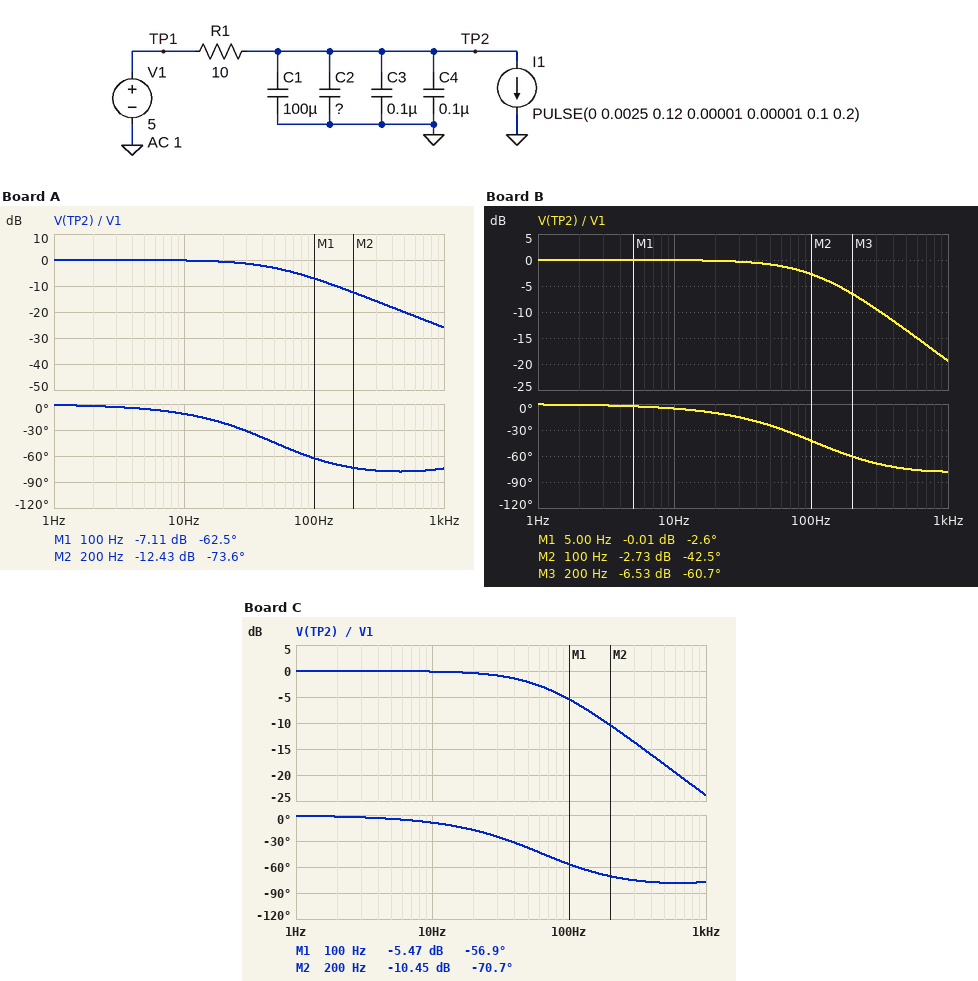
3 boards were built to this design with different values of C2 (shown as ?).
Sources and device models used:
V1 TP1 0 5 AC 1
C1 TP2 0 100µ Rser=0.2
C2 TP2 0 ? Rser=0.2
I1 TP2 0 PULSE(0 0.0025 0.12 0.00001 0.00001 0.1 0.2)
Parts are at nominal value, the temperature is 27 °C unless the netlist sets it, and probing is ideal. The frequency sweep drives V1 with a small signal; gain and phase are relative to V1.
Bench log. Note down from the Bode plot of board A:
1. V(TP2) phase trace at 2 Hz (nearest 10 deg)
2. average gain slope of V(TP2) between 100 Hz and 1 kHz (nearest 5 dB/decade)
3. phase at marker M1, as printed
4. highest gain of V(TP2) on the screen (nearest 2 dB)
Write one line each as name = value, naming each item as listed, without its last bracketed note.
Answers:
V(TP2) phase trace at 2 Hz = 0 deg
average gain slope of V(TP2) between 100 Hz and 1 kHz = -20 dB/decade
phase at marker M1, as printed = -62.5 deg
highest gain of V(TP2) on the screen = 0 dB
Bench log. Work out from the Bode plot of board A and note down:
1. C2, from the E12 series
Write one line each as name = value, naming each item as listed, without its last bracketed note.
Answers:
C2, from the E12 series = 220 µF
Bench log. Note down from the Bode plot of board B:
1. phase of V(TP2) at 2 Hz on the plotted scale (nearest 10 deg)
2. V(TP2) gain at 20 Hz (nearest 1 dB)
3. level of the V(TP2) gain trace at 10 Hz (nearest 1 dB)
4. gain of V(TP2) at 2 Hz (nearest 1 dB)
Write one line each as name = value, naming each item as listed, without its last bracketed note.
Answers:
phase of V(TP2) at 2 Hz on the plotted scale = 0 deg
V(TP2) gain at 20 Hz = 0 dB
level of the V(TP2) gain trace at 10 Hz = 0 dB
gain of V(TP2) at 2 Hz = 0 dB
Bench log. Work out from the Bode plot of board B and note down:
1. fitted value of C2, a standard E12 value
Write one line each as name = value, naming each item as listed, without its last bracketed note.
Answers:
fitted value of C2, a standard E12 value = 47 µF
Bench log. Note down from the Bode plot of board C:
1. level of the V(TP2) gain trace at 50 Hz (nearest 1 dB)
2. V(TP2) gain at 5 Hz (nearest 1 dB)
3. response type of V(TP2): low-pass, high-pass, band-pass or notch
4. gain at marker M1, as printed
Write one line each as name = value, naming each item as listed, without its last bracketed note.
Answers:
level of the V(TP2) gain trace at 50 Hz = -2 dB
V(TP2) gain at 5 Hz = 0 dB
response type of V(TP2): low-pass, high-pass, band-pass or notch = low-pass
gain at marker M1, as printed = -5.47 dB
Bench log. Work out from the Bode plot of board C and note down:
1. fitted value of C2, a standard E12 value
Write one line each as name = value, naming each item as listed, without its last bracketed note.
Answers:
fitted value of C2, a standard E12 value = 150 µF
